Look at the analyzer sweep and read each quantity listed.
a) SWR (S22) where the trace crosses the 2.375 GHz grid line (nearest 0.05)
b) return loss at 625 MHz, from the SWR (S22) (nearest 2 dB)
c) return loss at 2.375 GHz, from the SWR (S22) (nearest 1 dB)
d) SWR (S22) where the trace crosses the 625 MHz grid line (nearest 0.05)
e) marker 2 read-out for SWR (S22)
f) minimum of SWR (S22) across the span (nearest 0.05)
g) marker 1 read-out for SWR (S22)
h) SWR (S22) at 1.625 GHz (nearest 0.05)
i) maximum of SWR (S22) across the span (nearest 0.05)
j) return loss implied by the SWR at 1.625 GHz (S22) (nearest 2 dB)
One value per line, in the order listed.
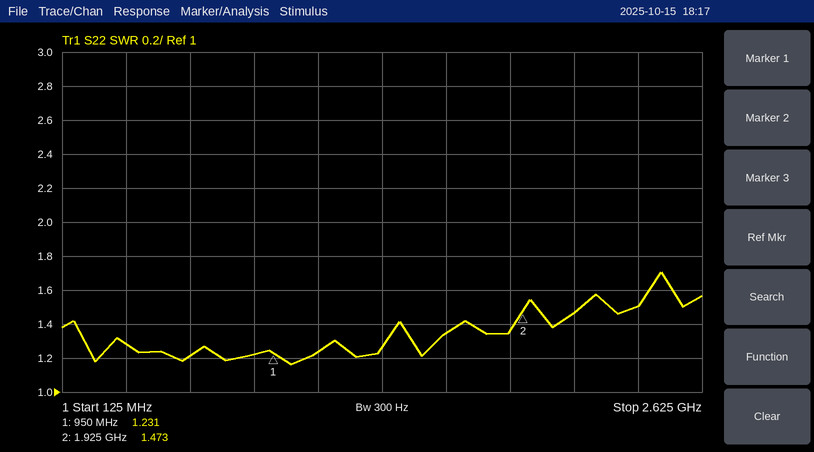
1.50
20 dB
14 dB
1.20
1.473
1.15
1.231
1.35
1.70
16 dB
